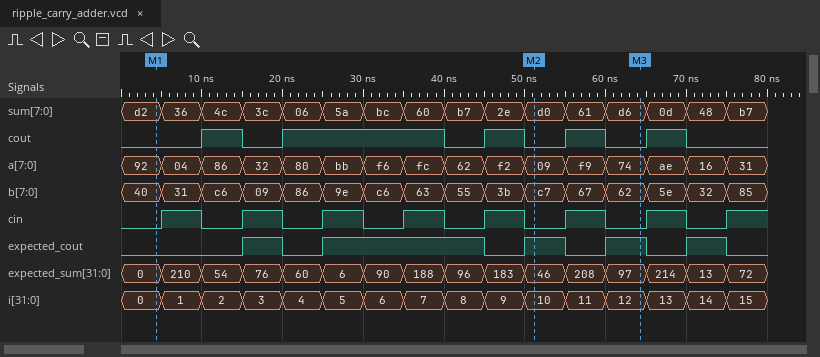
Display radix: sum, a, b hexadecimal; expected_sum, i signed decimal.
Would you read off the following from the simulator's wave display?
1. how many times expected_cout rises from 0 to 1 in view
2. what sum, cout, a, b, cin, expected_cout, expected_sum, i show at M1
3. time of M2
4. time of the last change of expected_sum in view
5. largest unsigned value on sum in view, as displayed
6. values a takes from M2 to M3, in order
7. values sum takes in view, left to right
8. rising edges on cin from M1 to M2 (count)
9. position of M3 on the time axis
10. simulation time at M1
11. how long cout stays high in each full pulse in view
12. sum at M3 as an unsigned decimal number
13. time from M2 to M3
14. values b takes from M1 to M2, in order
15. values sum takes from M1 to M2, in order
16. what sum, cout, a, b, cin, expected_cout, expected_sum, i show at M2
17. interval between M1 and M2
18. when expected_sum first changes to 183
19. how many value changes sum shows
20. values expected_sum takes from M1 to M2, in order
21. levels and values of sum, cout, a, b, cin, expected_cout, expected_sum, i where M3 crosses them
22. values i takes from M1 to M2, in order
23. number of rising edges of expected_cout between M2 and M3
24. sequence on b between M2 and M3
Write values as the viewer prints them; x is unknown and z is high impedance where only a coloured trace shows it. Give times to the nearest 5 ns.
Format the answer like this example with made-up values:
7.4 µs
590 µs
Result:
5
sum=d2, cout=0, a=92, b=40, cin=0, expected_cout=0, expected_sum=0, i=0
50 ns
75 ns
d6
09, f9, 74
d2, 36, 4c, 3c, 06, 5a, bc, 60, b7, 2e, d0, 61, d6, 0d, 48, b7
5
65 ns
5 ns
5 ns, 20 ns, 5 ns, 5 ns, 5 ns
214
15 ns
40, 31, c6, 09, 86, 9e, c6, 63, 55, 3b, c7
d2, 36, 4c, 3c, 06, 5a, bc, 60, b7, 2e, d0
sum=d0, cout=0, a=09, b=c7, cin=0, expected_cout=1, expected_sum=46, i=10
45 ns
45 ns
15
0, 210, 54, 76, 60, 6, 90, 188, 96, 183, 46
sum=d6, cout=0, a=74, b=62, cin=0, expected_cout=1, expected_sum=97, i=12
0, 1, 2, 3, 4, 5, 6, 7, 8, 9, 10
1
c7, 67, 62
